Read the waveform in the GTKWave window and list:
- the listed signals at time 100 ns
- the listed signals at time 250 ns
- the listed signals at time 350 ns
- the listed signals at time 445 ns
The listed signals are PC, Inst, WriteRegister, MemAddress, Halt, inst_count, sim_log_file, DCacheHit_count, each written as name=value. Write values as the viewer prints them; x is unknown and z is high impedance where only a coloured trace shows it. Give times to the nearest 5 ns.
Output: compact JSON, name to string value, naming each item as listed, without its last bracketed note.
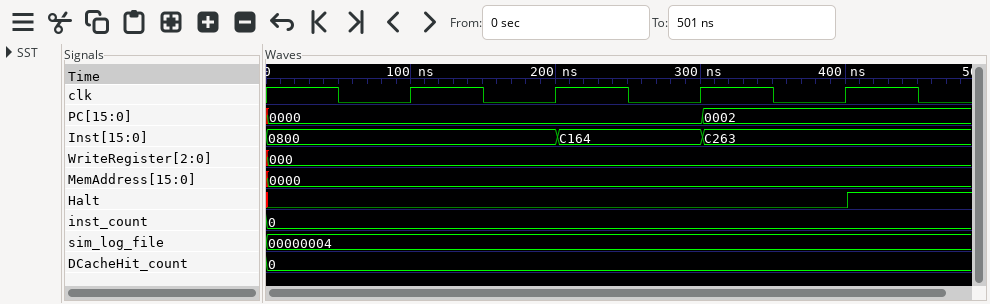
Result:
{"the listed signals at time 100 ns": "PC=0000, Inst=0800, WriteRegister=000, MemAddress=0000, Halt=0, inst_count=0, sim_log_file=00000004, DCacheHit_count=0", "the listed signals at time 250 ns": "PC=0000, Inst=C164, WriteRegister=000, MemAddress=0000, Halt=0, inst_count=0, sim_log_file=00000004, DCacheHit_count=0", "the listed signals at time 350 ns": "PC=0002, Inst=C263, WriteRegister=000, MemAddress=0000, Halt=0, inst_count=0, sim_log_file=00000004, DCacheHit_count=0", "the listed signals at time 445 ns": "PC=0002, Inst=C263, WriteRegister=000, MemAddress=0000, Halt=1, inst_count=0, sim_log_file=00000004, DCacheHit_count=0"}
